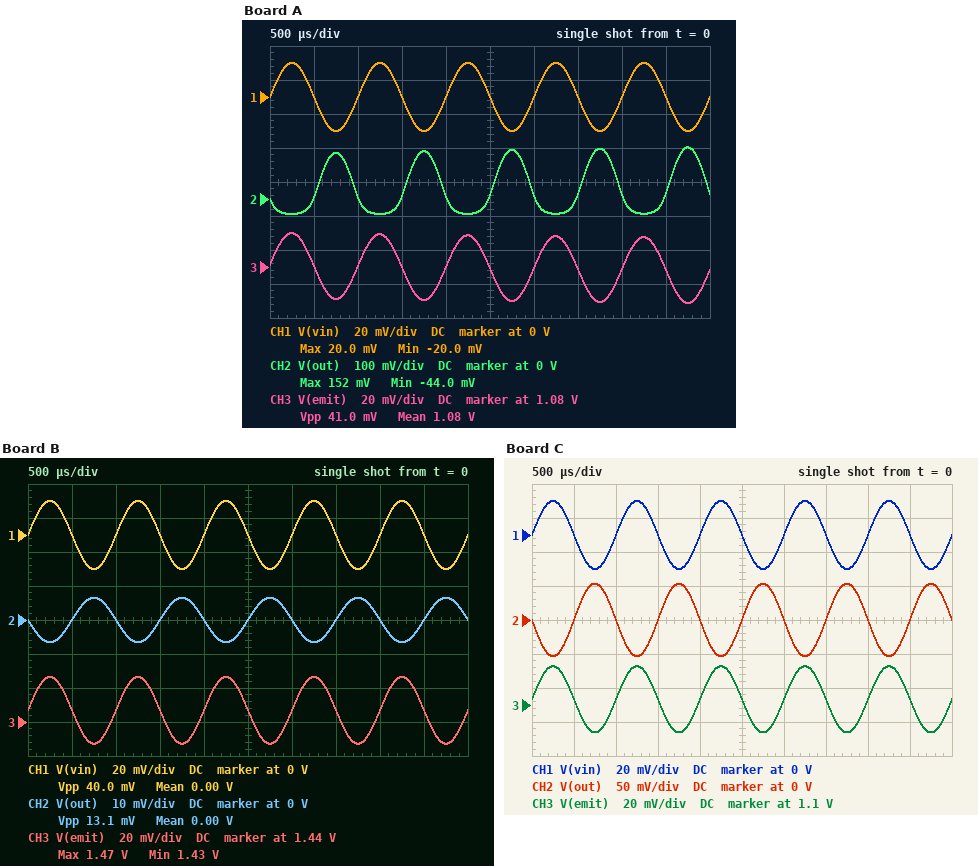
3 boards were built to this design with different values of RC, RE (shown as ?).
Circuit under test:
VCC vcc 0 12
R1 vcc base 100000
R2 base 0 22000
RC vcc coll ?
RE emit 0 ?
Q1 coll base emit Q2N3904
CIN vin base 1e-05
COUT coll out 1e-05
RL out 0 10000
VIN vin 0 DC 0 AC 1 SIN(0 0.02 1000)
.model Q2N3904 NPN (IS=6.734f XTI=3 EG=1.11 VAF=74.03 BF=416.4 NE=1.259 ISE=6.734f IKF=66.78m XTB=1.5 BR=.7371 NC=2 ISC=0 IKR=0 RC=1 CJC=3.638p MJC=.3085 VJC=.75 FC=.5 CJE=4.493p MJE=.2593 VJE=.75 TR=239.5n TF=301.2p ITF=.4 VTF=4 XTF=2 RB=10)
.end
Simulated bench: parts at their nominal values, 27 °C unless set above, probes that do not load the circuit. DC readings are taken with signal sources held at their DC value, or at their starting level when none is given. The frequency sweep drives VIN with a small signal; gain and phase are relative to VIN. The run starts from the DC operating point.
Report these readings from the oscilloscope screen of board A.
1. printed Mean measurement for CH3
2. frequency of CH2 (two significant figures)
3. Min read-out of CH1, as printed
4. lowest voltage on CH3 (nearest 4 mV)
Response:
1.08 V
1.0 kHz
-20.0 mV
1.060 V
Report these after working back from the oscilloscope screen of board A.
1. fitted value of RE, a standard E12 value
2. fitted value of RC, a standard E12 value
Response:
390 Ω
3.9 kΩ
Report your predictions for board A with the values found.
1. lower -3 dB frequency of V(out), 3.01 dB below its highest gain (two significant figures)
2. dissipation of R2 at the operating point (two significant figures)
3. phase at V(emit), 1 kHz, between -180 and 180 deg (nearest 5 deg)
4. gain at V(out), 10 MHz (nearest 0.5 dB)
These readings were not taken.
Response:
12 Hz
140 µW
0 deg
4.5 dB
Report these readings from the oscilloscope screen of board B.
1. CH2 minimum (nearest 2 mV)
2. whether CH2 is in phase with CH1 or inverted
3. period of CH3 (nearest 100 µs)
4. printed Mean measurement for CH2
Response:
-6 mV
inverted
1.0 ms
0.00 V
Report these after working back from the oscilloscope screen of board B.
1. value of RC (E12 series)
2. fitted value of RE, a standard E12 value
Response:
1 kΩ
2.7 kΩ
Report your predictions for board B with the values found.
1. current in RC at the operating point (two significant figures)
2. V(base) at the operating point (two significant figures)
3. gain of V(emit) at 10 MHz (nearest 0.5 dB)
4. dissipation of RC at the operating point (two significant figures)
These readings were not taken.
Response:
530 µA
2.1 V
0 dB
280 µW
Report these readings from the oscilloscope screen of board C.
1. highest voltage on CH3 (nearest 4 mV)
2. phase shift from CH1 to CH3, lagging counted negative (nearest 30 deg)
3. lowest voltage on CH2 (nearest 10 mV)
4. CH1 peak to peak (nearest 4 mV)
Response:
1.124 V
0 deg
-50 mV
40 mV
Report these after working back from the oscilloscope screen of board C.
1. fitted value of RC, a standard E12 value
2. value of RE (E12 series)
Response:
1 kΩ
330 Ω
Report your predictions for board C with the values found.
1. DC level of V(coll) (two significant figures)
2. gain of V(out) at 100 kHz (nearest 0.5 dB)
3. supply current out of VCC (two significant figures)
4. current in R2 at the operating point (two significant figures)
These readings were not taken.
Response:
8.7 V
8.5 dB
3.4 mA
82 µA
